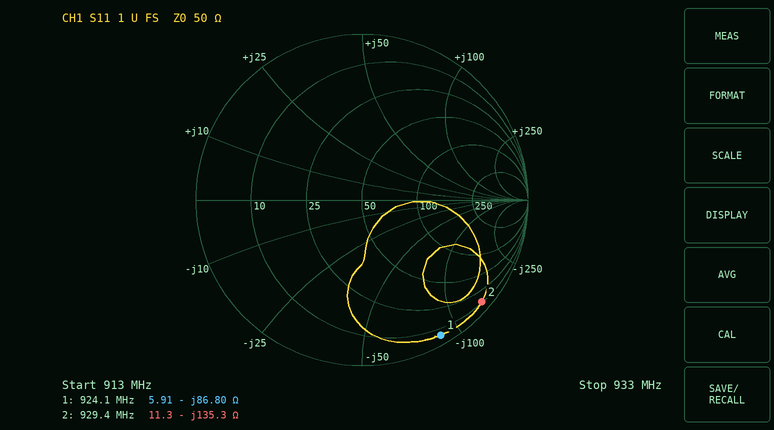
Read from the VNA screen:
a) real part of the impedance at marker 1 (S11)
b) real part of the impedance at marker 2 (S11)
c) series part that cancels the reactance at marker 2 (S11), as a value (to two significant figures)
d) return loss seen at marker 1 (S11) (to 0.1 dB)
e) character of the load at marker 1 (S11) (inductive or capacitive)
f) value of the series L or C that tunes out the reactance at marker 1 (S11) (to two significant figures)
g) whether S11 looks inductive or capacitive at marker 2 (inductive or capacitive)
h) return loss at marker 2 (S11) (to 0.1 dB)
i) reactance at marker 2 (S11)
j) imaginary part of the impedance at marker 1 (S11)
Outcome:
5.91 Ω
11.3 Ω
23 nH
0.5 dB
capacitive
15 nH
capacitive
0.5 dB
-135.3 Ω
-86.80 Ω
